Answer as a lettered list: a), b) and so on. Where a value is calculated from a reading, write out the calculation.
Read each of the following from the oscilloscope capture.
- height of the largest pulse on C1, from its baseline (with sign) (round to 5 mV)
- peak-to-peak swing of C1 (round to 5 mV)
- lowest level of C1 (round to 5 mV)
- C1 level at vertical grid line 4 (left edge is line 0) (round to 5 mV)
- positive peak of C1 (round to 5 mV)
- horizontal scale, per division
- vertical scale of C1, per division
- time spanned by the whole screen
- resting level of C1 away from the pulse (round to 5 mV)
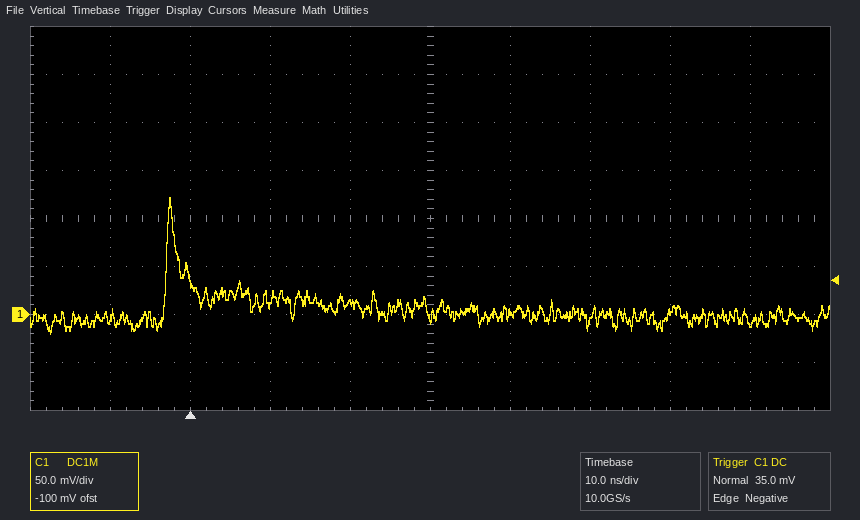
a) 120 mV − (0 mV) = +120 mV
b) 120 mV − (-20 mV) = 140 mV
c) -20 mV
d) 10 mV
e) 120 mV
f) 10 ns
g) 50 mV
h) 100 ns
i) 0 mV
